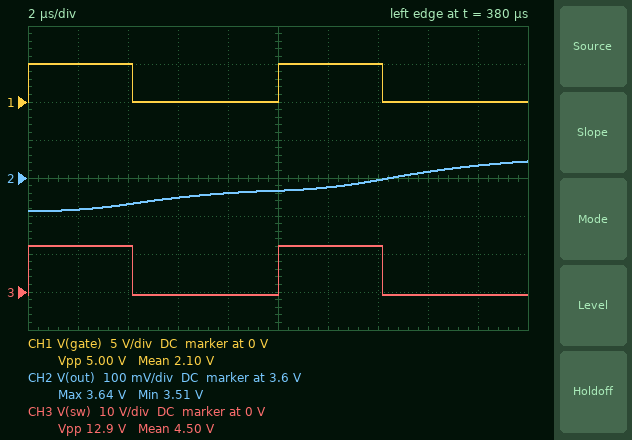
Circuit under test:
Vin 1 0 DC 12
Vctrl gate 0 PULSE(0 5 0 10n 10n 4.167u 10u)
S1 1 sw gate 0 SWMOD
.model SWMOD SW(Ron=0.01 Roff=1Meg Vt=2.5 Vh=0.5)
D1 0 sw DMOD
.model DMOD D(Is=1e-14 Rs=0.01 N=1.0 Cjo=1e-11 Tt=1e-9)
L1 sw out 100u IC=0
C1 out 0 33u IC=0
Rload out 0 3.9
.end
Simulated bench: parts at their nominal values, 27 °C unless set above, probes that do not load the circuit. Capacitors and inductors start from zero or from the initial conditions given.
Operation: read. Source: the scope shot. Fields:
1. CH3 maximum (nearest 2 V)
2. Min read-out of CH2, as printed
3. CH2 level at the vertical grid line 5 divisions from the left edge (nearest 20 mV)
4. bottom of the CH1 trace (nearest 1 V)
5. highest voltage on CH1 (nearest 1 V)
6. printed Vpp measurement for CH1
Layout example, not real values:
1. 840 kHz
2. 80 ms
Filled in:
1. 12 V
2. 3.51 V
3. 3.56 V
4. 0 V
5. 5 V
6. 5.00 V
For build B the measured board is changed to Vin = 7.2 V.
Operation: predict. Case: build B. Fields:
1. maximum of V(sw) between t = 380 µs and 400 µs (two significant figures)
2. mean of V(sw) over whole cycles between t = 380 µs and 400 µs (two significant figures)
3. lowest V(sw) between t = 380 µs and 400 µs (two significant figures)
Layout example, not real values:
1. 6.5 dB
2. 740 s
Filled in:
1. 7.2 V
2. 2.5 V
3. -830 mV
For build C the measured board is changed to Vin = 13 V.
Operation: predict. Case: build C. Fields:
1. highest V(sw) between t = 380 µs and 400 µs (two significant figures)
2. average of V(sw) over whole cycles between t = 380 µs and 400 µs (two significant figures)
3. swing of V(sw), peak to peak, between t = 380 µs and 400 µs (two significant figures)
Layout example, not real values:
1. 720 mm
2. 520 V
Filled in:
1. 13 V
2. 4.9 V
3. 14 V
